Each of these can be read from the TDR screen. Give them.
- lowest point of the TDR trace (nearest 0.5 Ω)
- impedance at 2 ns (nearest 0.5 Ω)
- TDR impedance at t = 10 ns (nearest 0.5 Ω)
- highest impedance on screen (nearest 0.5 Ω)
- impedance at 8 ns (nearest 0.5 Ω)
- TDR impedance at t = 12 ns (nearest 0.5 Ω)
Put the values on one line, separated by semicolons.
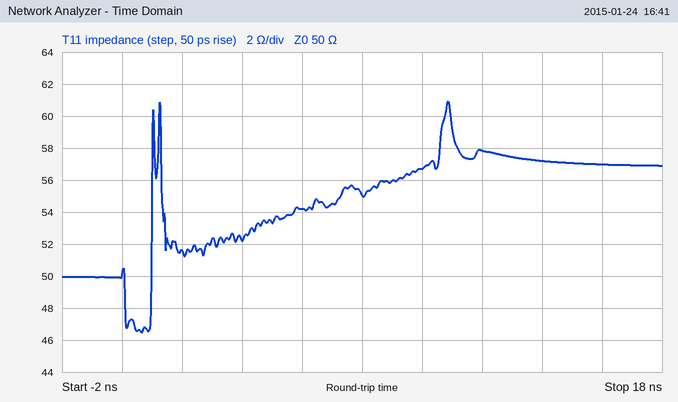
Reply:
46.5 Ω; 51.5 Ω; 56.5 Ω; 61.0 Ω; 55.0 Ω; 58.0 Ω
